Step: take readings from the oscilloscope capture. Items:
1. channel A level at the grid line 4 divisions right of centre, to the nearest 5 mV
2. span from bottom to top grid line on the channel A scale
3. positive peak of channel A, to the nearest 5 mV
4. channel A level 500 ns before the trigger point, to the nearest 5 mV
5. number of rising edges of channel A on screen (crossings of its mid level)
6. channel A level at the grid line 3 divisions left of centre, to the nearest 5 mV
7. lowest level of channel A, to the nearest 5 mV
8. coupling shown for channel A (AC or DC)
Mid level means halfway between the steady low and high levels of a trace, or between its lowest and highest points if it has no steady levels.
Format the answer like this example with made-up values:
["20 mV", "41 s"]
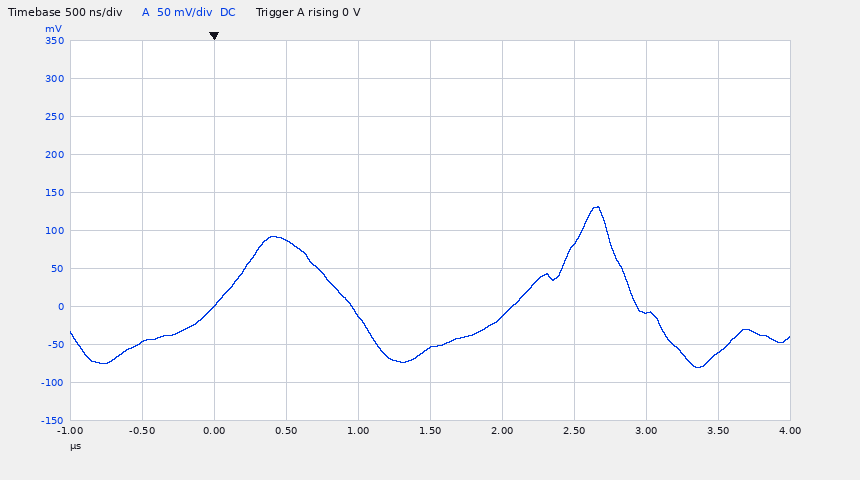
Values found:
["-60 mV", "500 mV", "130 mV", "-45 mV", "2", "0 mV", "-80 mV", "DC"]
